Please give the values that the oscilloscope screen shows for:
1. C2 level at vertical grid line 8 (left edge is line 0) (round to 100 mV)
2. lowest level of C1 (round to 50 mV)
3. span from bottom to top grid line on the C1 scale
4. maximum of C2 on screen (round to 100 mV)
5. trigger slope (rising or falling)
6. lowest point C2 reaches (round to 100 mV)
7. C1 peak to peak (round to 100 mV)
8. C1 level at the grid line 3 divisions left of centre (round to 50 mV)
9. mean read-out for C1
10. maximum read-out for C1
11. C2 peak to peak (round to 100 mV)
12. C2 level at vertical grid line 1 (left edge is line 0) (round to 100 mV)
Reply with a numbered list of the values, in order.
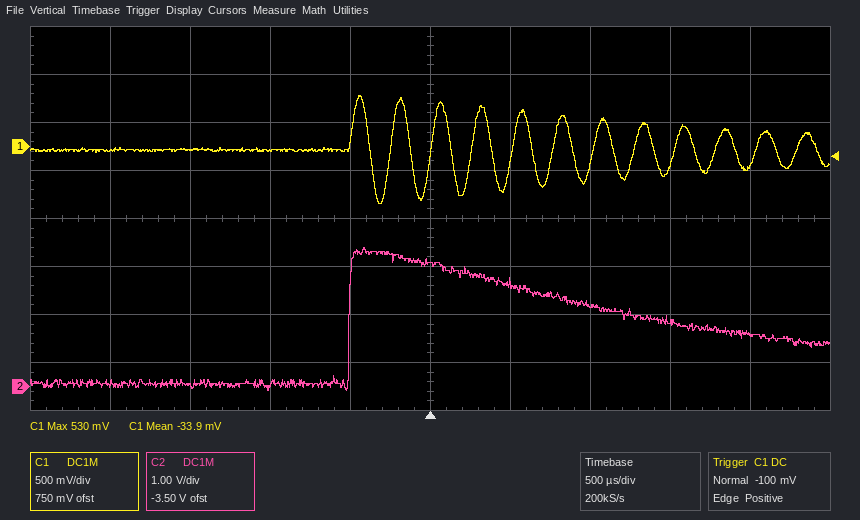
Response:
1. 1.4 V
2. -600 mV
3. 4 V
4. 2.9 V
5. rising
6. -100 mV
7. 1.10 V
8. -50 mV
9. -33.9 mV
10. 530 mV
11. 3.0 V
12. 100 mV
